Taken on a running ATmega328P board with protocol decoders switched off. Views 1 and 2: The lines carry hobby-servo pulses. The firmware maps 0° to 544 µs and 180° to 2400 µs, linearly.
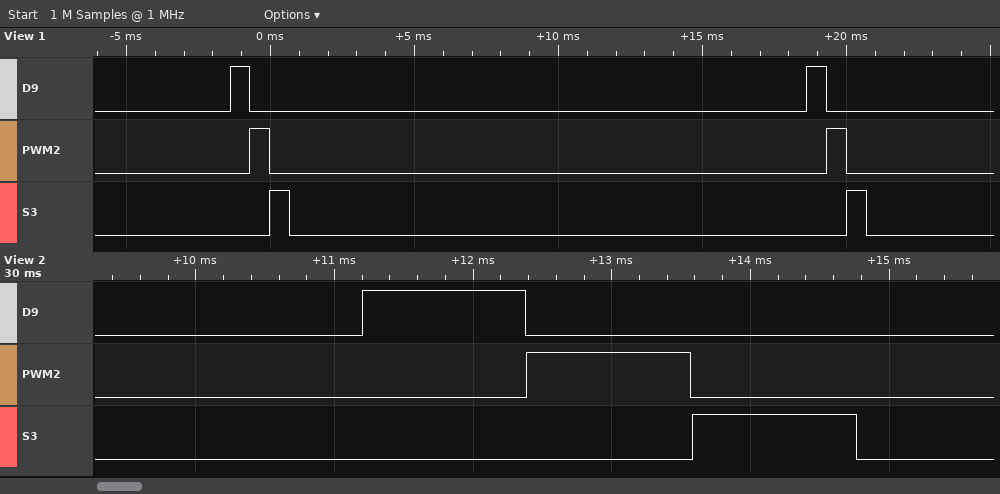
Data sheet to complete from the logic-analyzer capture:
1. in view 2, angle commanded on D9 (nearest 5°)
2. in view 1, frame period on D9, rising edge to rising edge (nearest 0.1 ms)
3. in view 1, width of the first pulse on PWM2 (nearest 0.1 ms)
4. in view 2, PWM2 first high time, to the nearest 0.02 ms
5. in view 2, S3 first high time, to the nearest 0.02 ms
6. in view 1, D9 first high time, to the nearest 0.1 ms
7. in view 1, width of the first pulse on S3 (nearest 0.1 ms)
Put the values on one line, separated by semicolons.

60°; 20.0 ms; 0.7 ms; 1.18 ms; 1.18 ms; 0.7 ms; 0.7 ms
